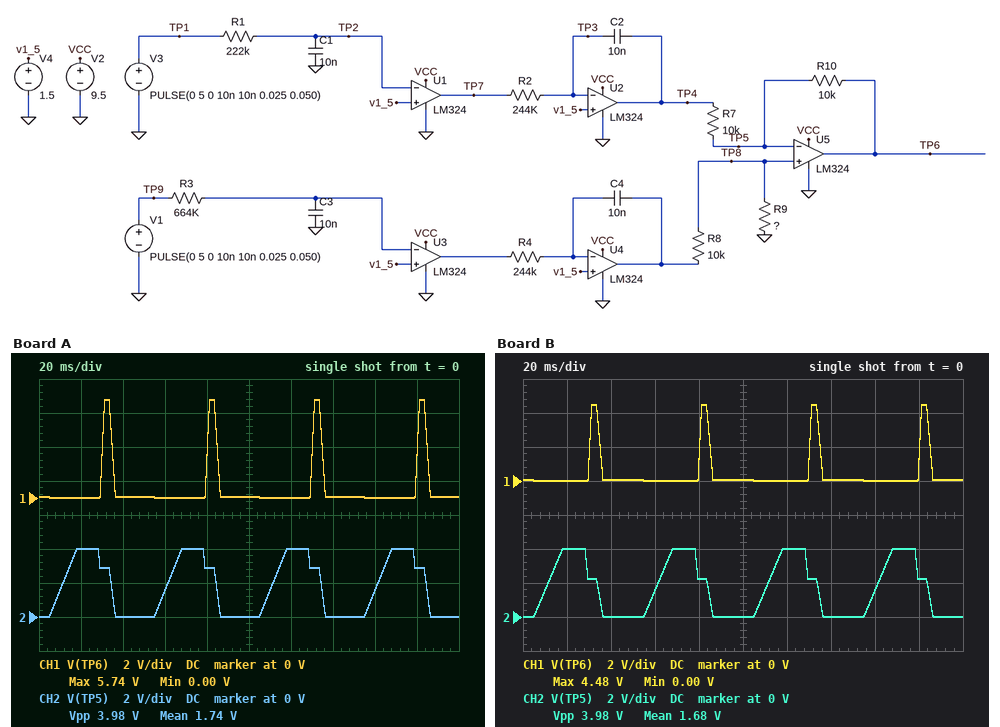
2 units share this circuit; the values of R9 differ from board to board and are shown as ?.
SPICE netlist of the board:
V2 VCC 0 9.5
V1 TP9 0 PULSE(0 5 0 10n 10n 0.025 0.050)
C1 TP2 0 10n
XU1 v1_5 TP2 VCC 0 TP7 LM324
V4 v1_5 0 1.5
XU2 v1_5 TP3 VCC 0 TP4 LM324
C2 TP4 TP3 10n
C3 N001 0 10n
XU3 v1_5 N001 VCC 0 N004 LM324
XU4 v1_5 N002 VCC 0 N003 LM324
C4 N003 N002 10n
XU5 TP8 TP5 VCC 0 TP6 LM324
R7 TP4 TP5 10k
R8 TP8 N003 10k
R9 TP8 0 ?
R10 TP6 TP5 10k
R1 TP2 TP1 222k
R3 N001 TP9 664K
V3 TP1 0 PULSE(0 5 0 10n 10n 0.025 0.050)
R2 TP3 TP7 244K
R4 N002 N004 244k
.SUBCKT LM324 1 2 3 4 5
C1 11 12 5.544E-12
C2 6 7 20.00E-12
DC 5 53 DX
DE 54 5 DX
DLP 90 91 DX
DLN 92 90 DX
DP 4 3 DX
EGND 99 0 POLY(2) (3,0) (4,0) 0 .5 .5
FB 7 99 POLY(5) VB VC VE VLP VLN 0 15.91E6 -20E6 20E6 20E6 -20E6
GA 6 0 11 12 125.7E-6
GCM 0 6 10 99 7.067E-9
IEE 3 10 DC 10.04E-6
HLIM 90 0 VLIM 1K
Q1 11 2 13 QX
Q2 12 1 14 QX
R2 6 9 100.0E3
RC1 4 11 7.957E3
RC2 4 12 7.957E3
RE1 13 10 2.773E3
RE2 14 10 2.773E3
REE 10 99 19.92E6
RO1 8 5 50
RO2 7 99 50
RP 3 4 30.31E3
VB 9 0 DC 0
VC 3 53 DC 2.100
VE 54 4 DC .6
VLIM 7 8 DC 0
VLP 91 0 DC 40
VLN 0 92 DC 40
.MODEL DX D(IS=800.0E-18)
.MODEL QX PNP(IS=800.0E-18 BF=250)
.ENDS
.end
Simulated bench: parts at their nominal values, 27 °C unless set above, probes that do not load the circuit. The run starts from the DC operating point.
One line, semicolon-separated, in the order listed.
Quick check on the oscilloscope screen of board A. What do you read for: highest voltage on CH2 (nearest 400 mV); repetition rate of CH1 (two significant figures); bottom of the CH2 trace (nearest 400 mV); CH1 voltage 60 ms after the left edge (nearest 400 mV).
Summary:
4.0 V; 20 Hz; 0 V; 0 V
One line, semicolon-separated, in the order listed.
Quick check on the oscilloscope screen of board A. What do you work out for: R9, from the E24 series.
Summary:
5.6 kΩ
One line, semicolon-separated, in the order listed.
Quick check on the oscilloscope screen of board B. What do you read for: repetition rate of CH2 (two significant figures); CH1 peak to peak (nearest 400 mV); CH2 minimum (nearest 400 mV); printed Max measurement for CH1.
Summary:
20 Hz; 4.4 V; 0 V; 4.48 V
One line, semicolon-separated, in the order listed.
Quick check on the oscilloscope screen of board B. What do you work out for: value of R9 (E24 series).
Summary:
3.9 kΩ
